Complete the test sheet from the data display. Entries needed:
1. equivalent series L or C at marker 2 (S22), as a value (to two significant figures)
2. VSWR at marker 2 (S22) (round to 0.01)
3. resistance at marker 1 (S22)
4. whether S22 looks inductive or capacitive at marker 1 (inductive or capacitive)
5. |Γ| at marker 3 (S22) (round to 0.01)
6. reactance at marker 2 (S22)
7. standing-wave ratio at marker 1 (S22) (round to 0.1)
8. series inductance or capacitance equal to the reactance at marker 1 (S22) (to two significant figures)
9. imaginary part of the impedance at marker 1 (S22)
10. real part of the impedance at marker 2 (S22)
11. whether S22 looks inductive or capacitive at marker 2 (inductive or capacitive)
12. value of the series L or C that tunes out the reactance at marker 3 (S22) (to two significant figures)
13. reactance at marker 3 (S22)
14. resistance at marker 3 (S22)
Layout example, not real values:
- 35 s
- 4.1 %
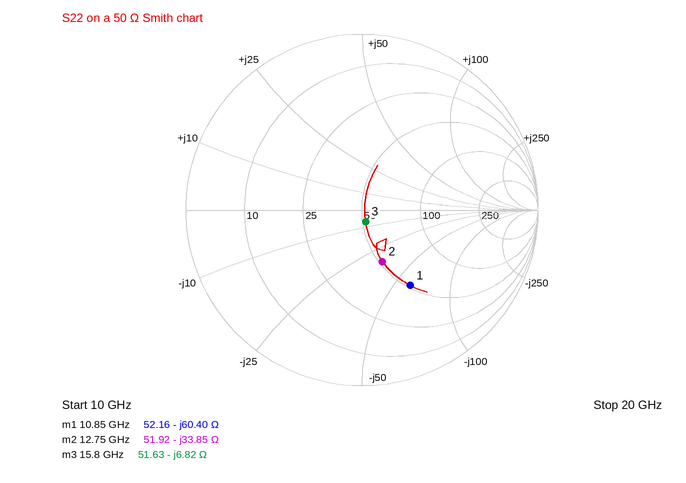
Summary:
- 370 fF
- 1.92
- 52.16 Ω
- capacitive
- 0.07
- -33.85 Ω
- 3.1
- 240 fF
- -60.40 Ω
- 51.92 Ω
- capacitive
- 69 pH
- -6.82 Ω
- 51.63 Ω
